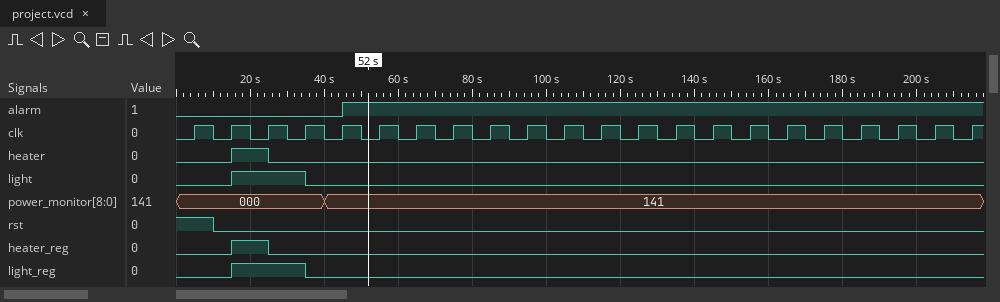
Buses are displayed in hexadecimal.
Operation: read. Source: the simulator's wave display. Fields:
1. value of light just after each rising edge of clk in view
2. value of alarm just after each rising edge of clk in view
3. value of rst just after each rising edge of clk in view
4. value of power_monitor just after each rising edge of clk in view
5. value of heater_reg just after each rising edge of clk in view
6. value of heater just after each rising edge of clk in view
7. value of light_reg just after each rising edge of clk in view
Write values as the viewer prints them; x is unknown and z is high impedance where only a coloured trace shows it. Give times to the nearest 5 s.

0 1 1 0 0 0 0 0 0 0 0 0 0 0 0 0 0 0 0 0 0 0
0 0 0 0 1 1 1 1 1 1 1 1 1 1 1 1 1 1 1 1 1 1
1 0 0 0 0 0 0 0 0 0 0 0 0 0 0 0 0 0 0 0 0 0
000, 000, 000, 000, 141, 141, 141, 141, 141, 141, 141, 141, 141, 141, 141, 141, 141, 141, 141, 141, 141, 141
0 1 0 0 0 0 0 0 0 0 0 0 0 0 0 0 0 0 0 0 0 0
0 1 0 0 0 0 0 0 0 0 0 0 0 0 0 0 0 0 0 0 0 0
0 1 1 0 0 0 0 0 0 0 0 0 0 0 0 0 0 0 0 0 0 0
